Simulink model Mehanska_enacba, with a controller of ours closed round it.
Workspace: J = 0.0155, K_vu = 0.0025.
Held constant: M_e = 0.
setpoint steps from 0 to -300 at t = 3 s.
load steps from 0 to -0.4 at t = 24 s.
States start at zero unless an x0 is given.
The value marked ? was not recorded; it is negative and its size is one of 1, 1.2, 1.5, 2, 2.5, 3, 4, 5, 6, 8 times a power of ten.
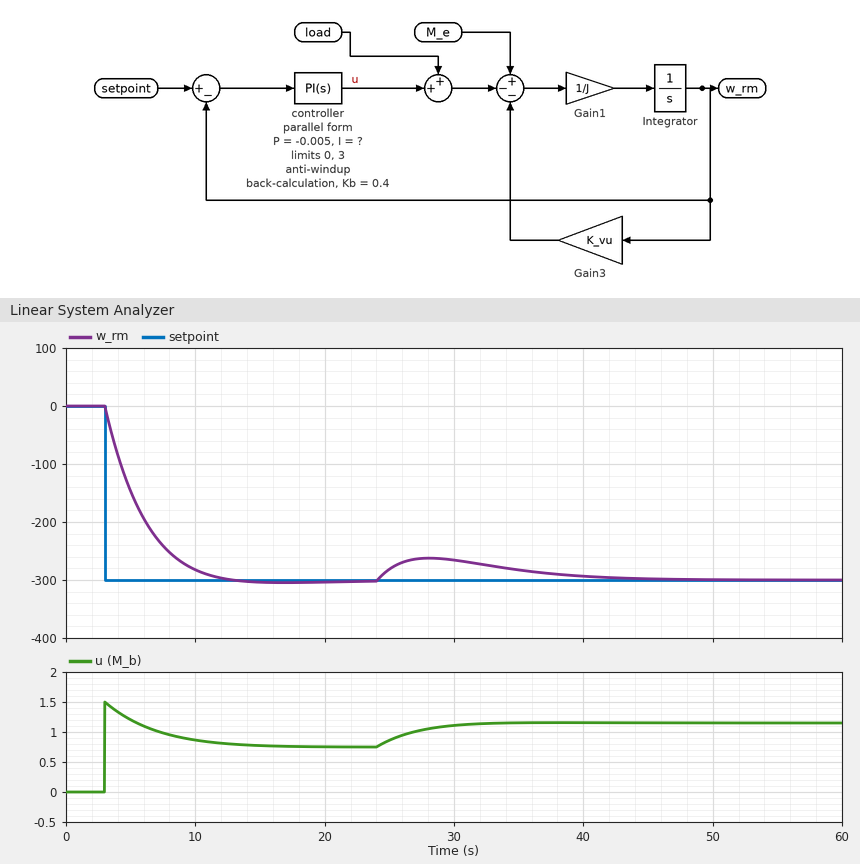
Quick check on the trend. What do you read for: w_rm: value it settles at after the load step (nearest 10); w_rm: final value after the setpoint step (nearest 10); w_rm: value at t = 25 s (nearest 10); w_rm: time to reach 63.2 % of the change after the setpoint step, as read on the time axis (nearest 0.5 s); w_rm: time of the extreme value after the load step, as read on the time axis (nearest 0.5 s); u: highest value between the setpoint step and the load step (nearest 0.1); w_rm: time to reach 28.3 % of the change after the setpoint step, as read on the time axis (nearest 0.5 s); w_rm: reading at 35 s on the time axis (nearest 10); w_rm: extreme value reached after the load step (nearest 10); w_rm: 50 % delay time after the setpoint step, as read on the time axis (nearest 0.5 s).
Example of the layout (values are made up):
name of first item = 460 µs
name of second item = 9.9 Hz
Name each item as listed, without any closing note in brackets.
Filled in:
w_rm: value it settles at after the load step = -300
w_rm: final value after the setpoint step = -300
w_rm: value at t = 25 s = -280
w_rm: time to reach 63.2 % of the change after the setpoint step, as read on the time axis = 6.0 s
w_rm: time of the extreme value after the load step, as read on the time axis = 28.0 s
u: highest value between the setpoint step and the load step = 1.5
w_rm: time to reach 28.3 % of the change after the setpoint step, as read on the time axis = 4.0 s
w_rm: reading at 35 s on the time axis = -280
w_rm: extreme value reached after the load step = -260
w_rm: 50 % delay time after the setpoint step, as read on the time axis = 5.0 s
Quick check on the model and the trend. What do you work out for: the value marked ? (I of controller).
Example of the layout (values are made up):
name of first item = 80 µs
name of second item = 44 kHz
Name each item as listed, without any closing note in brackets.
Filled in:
the value marked ? = -0.001
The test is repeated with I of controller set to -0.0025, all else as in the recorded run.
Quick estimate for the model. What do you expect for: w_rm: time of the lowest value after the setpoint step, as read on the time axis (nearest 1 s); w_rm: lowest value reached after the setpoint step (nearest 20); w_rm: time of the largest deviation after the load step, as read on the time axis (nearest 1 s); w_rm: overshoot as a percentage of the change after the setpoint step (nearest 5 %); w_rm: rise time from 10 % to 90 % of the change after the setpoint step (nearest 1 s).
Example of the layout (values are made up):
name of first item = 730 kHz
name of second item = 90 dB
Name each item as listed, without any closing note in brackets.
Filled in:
w_rm: time of the lowest value after the setpoint step, as read on the time axis = 10 s
w_rm: lowest value reached after the setpoint step = -340
w_rm: time of the largest deviation after the load step, as read on the time axis = 27 s
w_rm: overshoot as a percentage of the change after the setpoint step = 15 %
w_rm: rise time from 10 % to 90 % of the change after the setpoint step = 3 s
